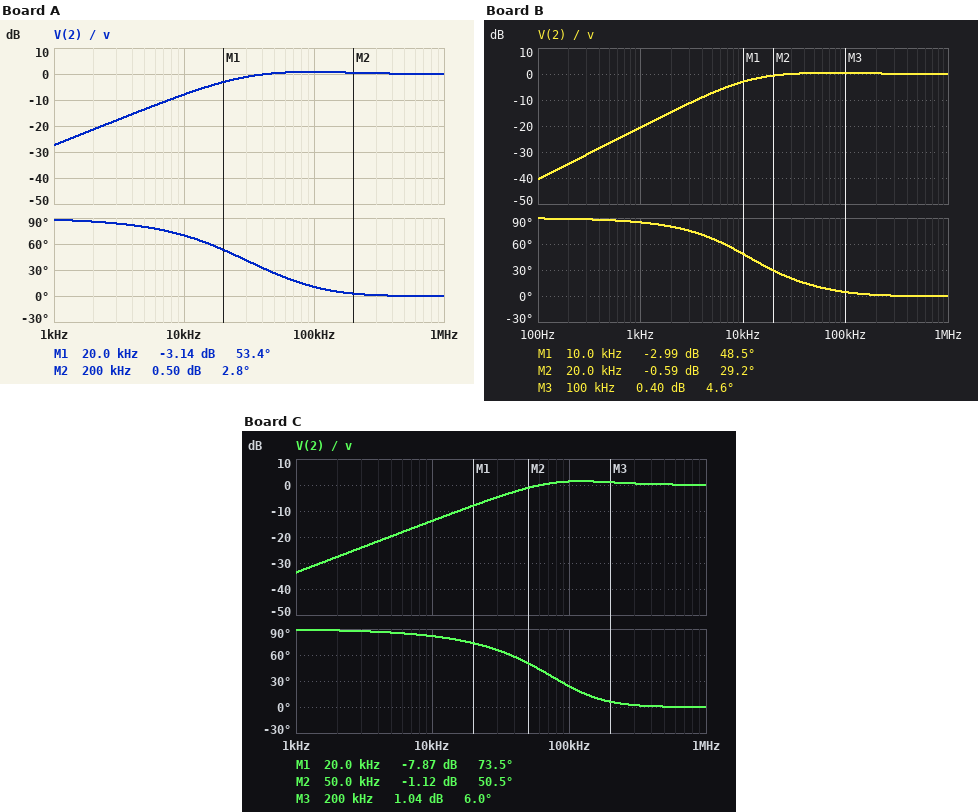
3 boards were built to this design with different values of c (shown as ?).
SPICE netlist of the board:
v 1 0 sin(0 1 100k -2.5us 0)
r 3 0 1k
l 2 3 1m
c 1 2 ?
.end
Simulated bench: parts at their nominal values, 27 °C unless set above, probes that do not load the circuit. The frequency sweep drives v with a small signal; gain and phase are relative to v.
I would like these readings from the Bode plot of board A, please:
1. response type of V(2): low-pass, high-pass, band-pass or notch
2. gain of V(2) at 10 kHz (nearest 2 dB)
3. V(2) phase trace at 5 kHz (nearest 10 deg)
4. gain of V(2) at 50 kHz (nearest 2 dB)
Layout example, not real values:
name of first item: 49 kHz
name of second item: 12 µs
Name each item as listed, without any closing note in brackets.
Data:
response type of V(2): low-pass, high-pass, band-pass or notch: high-pass
gain of V(2) at 10 kHz: -8 dB
V(2) phase trace at 5 kHz: 80 deg
gain of V(2) at 50 kHz: 0 dB
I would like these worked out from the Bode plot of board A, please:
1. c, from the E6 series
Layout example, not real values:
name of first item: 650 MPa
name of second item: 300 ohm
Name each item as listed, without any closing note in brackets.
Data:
c, from the E6 series: 6.8 nF
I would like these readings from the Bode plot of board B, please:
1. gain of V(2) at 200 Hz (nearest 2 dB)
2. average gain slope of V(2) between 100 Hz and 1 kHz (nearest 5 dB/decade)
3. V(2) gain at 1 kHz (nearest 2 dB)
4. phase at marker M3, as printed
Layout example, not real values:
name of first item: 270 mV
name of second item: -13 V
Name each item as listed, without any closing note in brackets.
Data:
gain of V(2) at 200 Hz: -34 dB
average gain slope of V(2) between 100 Hz and 1 kHz: 20 dB/decade
V(2) gain at 1 kHz: -20 dB
phase at marker M3, as printed: 4.6 deg
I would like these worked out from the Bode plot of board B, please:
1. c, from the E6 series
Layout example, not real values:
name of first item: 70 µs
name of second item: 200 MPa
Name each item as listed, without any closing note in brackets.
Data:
c, from the E6 series: 15 nF
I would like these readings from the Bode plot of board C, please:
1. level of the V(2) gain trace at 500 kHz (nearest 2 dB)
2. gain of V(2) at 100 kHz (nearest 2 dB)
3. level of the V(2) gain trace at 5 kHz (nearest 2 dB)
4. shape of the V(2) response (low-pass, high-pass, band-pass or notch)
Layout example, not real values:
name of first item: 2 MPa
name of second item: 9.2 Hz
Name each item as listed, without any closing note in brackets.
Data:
level of the V(2) gain trace at 500 kHz: 0 dB
gain of V(2) at 100 kHz: 2 dB
level of the V(2) gain trace at 5 kHz: -20 dB
shape of the V(2) response: high-pass
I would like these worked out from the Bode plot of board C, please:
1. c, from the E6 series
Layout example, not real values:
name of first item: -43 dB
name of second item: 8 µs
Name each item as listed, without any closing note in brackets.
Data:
c, from the E6 series: 3.3 nF
